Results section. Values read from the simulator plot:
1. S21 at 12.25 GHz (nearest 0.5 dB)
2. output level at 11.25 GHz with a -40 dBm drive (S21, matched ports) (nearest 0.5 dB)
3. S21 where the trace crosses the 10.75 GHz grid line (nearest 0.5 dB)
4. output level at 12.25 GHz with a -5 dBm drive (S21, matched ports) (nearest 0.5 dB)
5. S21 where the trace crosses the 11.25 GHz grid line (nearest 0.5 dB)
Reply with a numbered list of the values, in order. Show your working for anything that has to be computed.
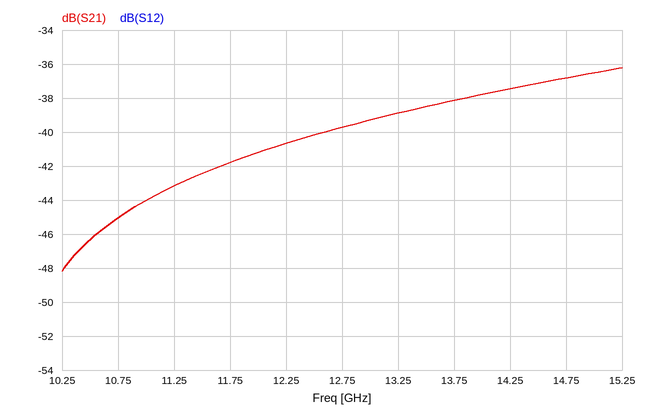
1. -40.5 dB
2. -40 dBm + (-43.0 dB) = -83.0 dBm
3. -45.0 dB
4. -5 dBm + (-40.5 dB) = -45.5 dBm
5. -43.0 dB
